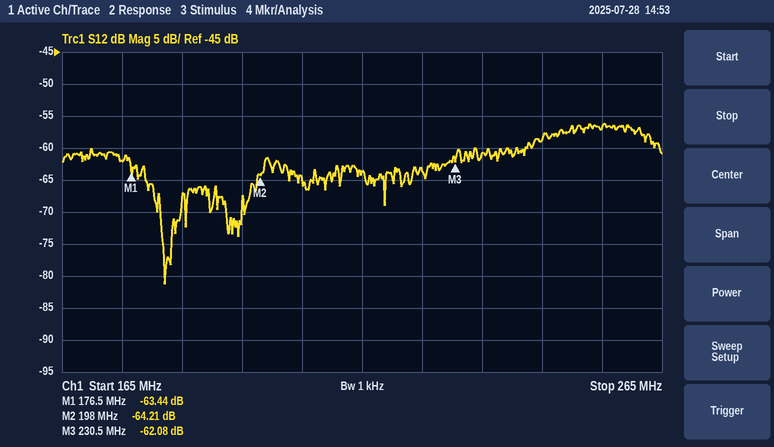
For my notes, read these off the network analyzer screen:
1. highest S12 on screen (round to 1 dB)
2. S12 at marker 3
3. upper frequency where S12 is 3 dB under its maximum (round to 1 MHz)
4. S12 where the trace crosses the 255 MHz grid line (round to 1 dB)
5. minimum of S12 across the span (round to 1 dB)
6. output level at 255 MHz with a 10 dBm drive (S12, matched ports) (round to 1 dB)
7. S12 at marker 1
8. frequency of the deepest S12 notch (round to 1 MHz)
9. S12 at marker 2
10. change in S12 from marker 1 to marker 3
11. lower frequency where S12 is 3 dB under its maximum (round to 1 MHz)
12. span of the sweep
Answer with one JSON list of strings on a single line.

["-56 dB", "-62.08 dB", "263 MHz", "-57 dB", "-81 dB", "-47 dBm", "-63.44 dB", "182 MHz", "-64.21 dB", "1.36 dB", "244 MHz", "100 MHz"]
